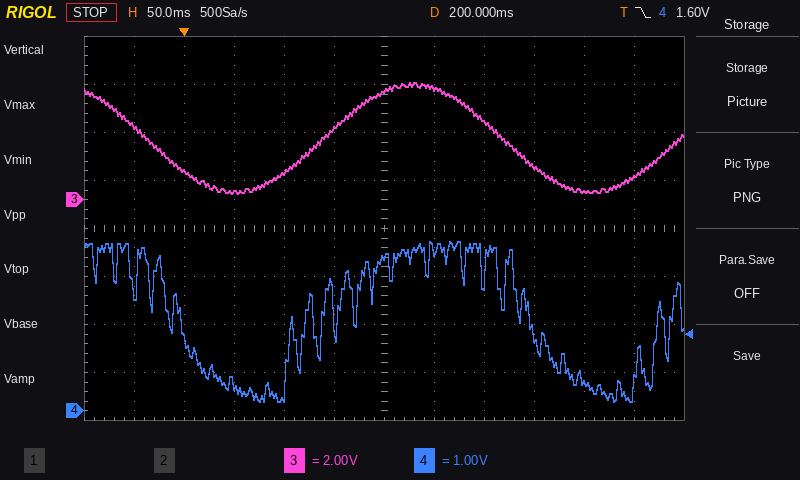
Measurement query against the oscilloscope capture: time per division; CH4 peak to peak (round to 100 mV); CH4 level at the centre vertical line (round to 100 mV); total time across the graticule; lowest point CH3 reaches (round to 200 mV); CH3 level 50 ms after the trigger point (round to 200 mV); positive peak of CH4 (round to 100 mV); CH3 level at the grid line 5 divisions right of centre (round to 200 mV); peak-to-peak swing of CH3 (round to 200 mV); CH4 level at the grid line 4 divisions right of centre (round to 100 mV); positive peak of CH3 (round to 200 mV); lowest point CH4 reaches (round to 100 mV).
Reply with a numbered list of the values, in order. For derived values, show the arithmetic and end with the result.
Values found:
1. 50 ms
2. 3.5 V − (200 mV) = 3.3 V
3. 3.2 V
4. 600 ms
5. 200 mV
6. 400 mV
7. 3.5 V
8. 1.0 V
9. 4.8 V − (200 mV) = 4.6 V
10. 600 mV
11. 4.8 V
12. 200 mV
